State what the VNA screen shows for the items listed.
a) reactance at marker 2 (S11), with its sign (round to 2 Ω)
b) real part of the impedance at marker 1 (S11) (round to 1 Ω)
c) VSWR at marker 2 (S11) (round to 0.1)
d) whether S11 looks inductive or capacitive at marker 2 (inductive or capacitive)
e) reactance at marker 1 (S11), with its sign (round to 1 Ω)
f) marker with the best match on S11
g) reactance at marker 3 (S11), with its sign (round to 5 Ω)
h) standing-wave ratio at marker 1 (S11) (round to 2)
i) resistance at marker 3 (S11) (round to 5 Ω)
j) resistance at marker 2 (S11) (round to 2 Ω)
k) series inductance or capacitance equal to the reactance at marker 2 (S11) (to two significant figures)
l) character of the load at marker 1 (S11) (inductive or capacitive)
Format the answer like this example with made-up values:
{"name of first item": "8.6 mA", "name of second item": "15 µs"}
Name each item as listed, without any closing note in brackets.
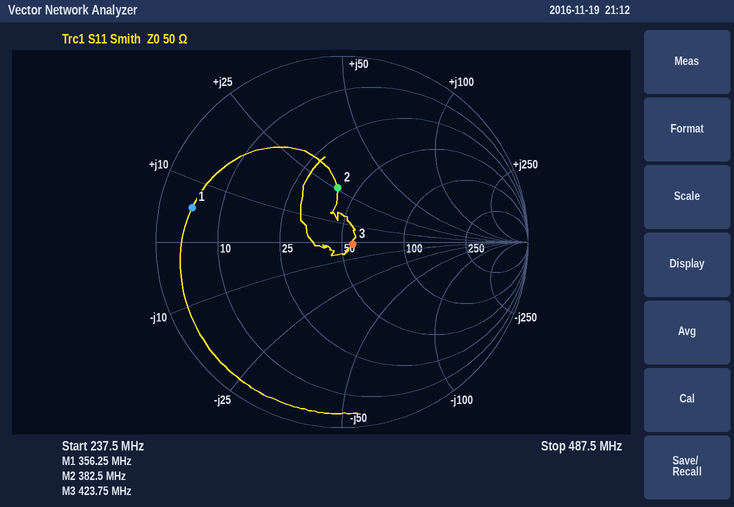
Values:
{"reactance at marker 2 (S11), with its sign": "+26 Ω", "real part of the impedance at marker 1 (S11)": "5 Ω", "VSWR at marker 2 (S11)": "1.8", "whether S11 looks inductive or capacitive at marker 2": "inductive", "reactance at marker 1 (S11), with its sign": "+6 Ω", "marker with the best match on S11": "marker 3", "reactance at marker 3 (S11), with its sign": "0 Ω", "standing-wave ratio at marker 1 (S11)": "10", "resistance at marker 3 (S11)": "55 Ω", "resistance at marker 2 (S11)": "40 Ω", "series inductance or capacitance equal to the reactance at marker 2 (S11)": "11 nH", "character of the load at marker 1 (S11)": "inductive"}
